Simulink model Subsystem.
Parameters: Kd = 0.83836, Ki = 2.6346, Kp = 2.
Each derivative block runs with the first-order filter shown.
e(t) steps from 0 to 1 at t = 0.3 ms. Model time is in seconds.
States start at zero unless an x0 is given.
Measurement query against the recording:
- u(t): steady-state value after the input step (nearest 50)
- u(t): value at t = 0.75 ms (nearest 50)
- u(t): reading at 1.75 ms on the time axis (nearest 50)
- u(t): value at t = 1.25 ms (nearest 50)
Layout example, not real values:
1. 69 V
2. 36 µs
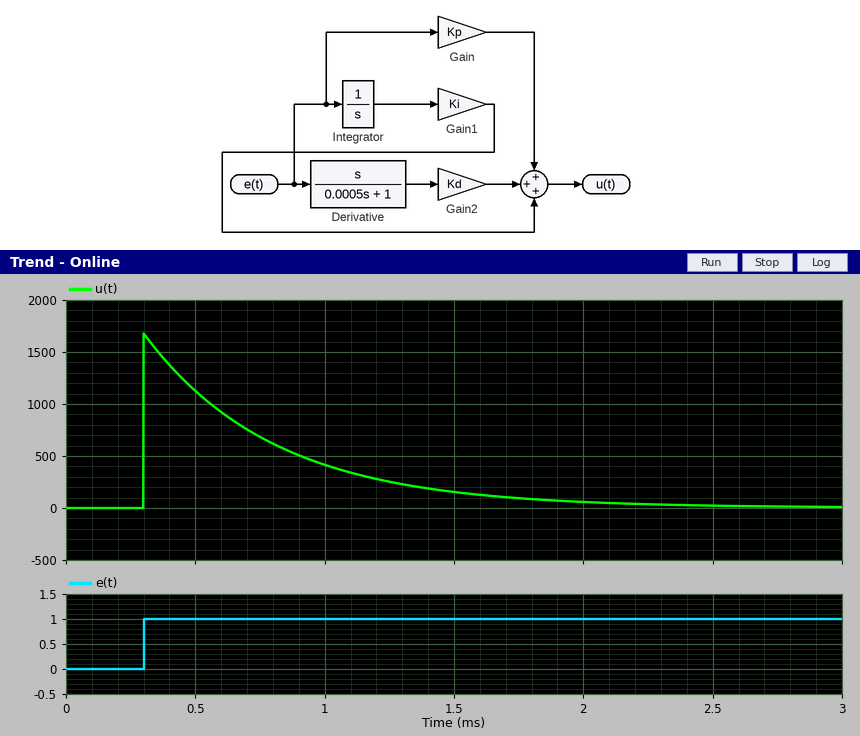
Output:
1. 0
2. 700
3. 100
4. 250
